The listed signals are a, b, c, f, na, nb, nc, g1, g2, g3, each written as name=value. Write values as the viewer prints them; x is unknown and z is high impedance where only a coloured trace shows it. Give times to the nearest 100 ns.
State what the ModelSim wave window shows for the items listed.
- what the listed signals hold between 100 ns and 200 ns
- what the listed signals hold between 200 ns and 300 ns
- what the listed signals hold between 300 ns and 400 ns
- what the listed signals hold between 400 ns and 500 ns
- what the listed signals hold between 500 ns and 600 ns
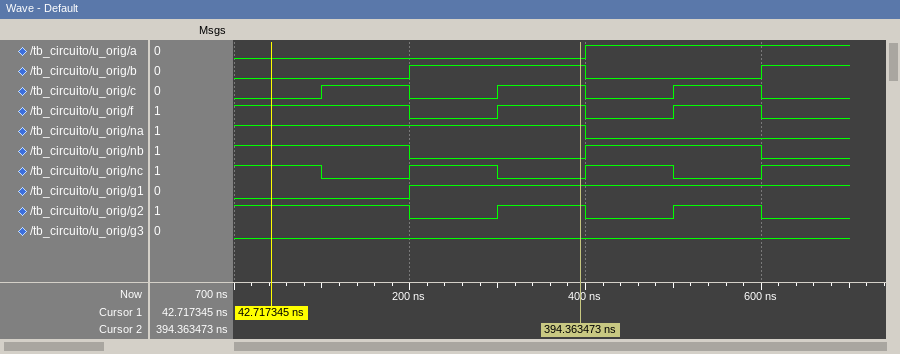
a=0, b=0, c=1, f=1, na=1, nb=1, nc=0, g1=0, g2=1, g3=0
a=0, b=1, c=0, f=0, na=1, nb=0, nc=1, g1=1, g2=0, g3=0
a=0, b=1, c=1, f=1, na=1, nb=0, nc=0, g1=1, g2=1, g3=0
a=1, b=0, c=0, f=0, na=0, nb=1, nc=1, g1=1, g2=0, g3=0
a=1, b=0, c=1, f=1, na=0, nb=1, nc=0, g1=1, g2=1, g3=0
